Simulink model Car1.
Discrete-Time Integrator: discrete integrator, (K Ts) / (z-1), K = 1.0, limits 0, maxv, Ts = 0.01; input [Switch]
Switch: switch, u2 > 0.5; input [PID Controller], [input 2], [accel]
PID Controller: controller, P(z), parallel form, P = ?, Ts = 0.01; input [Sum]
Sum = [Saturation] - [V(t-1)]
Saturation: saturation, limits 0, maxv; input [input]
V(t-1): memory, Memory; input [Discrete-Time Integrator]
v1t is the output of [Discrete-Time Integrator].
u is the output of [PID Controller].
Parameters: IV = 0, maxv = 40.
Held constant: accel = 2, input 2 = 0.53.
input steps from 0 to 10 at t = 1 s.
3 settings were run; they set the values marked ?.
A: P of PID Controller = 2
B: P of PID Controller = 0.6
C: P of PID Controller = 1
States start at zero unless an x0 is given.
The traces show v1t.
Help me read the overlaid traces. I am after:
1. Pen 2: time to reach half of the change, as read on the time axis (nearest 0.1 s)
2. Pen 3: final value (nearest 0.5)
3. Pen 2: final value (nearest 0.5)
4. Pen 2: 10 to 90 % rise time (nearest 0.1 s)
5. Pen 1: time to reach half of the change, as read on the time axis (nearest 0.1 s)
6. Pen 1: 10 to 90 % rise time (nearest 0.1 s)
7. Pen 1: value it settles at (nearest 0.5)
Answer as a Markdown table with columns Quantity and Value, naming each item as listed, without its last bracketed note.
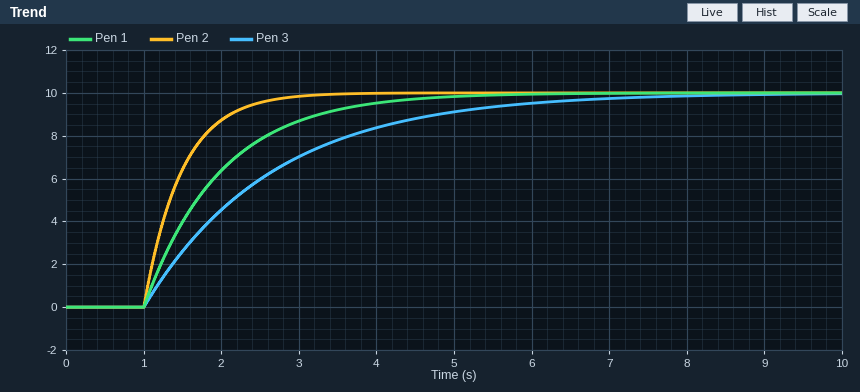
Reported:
| Quantity | Value |
|---|---|
| Pen 2: time to reach half of the change, as read on the time axis | 1.3 s |
| Pen 3: final value | 10.0 |
| Pen 2: final value | 10.0 |
| Pen 2: 10 to 90 % rise time | 1.1 s |
| Pen 1: time to reach half of the change, as read on the time axis | 1.7 s |
| Pen 1: 10 to 90 % rise time | 2.2 s |
| Pen 1: value it settles at | 10.0 |
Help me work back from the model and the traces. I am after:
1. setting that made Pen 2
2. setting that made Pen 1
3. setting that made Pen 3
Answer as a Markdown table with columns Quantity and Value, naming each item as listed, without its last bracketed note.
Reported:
| Quantity | Value |
|---|---|
| setting that made Pen 2 | A |
| setting that made Pen 1 | C |
| setting that made Pen 3 | B |
